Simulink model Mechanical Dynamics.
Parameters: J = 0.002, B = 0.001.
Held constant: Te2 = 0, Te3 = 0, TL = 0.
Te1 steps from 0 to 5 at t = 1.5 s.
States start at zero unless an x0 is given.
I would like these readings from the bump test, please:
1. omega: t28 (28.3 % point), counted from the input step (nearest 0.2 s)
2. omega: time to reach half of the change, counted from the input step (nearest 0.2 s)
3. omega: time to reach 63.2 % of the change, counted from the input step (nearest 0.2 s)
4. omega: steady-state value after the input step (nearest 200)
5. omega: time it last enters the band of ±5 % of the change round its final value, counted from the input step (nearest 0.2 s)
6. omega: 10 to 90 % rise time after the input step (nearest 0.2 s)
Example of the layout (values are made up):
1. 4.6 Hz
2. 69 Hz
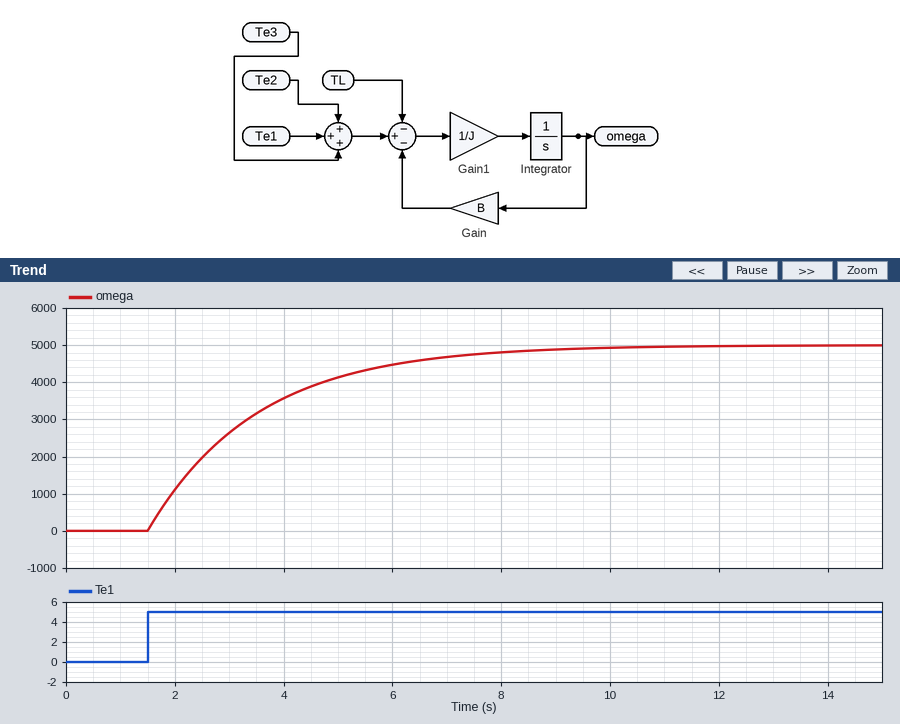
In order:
1. 0.6 s
2. 1.4 s
3. 2.0 s
4. 5000
5. 6.0 s
6. 4.4 s
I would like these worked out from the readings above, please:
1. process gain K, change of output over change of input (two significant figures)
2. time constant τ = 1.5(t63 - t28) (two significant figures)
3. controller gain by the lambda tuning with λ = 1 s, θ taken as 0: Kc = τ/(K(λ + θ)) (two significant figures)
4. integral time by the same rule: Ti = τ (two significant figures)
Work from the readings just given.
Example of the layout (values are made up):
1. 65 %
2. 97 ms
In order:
1. 1000
2. 2.1 s
3. 0.0021
4. 2.1 s
